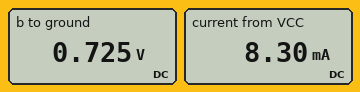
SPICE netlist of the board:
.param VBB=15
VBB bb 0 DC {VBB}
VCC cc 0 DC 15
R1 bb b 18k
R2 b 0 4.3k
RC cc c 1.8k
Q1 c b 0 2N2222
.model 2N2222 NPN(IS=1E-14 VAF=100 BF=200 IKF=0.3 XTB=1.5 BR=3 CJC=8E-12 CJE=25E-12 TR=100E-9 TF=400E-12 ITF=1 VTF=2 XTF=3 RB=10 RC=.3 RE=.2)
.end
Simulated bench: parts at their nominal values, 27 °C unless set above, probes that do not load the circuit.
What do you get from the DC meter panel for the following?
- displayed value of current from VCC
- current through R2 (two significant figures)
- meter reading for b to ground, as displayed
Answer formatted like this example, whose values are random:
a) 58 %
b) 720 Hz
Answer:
a) 8.30 mA
b) 170 µA
c) 0.725 V
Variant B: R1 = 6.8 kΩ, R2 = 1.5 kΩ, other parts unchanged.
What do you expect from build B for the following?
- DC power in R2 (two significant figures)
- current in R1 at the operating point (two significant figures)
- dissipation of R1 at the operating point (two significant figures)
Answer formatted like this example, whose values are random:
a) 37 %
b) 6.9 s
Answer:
a) 370 µW
b) 2.1 mA
c) 30 mW
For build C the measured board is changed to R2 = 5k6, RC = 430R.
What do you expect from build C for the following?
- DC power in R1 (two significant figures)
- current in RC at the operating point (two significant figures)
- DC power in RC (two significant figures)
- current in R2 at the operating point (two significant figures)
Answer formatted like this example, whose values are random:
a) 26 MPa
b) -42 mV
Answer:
a) 11 mW
b) 35 mA
c) 520 mW
d) 140 µA
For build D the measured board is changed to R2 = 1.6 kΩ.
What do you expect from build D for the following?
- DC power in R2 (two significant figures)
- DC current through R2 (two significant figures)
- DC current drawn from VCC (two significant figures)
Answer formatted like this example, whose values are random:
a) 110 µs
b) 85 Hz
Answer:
a) 320 µW
b) 450 µA
c) 8.3 mA
